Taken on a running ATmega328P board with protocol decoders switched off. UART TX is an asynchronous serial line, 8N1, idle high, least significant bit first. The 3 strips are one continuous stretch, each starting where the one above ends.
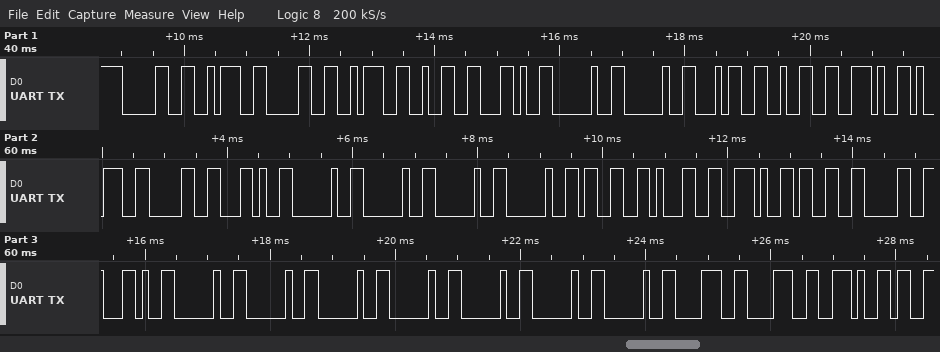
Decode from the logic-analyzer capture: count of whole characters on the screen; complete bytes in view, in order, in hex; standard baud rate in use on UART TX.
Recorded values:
34
30 3A 30 3A 32 2C 20 20 34 32 2E 39 30 2C 20 20 20 20 33 31 2E 33 30 2C 20 20 20 20 20 20 20 38 38 2E
9600 baud
